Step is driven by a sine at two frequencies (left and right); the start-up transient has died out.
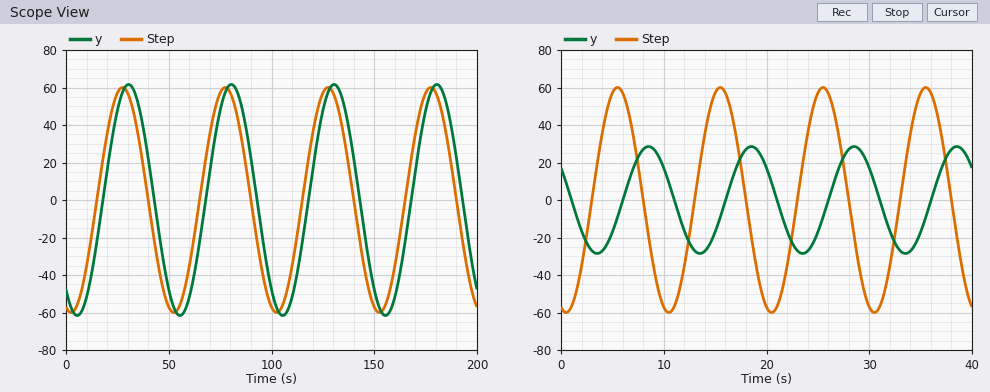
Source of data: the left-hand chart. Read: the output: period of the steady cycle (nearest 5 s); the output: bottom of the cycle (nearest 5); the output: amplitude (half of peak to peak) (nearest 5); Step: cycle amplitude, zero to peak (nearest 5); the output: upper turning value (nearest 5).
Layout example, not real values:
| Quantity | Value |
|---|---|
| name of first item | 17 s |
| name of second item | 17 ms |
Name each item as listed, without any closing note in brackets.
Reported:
| Quantity | Value |
|---|---|
| the output: period of the steady cycle | 50 s |
| the output: bottom of the cycle | -60 |
| the output: amplitude (half of peak to peak) | 60 |
| Step: cycle amplitude, zero to peak | 60 |
| the output: upper turning value | 60 |
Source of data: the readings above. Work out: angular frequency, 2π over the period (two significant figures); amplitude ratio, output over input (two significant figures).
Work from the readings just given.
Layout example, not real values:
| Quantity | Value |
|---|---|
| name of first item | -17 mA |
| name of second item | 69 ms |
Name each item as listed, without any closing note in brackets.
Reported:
| Quantity | Value |
|---|---|
| angular frequency, 2π over the period | 0.13 rad/s |
| amplitude ratio, output over input | 1.0 |
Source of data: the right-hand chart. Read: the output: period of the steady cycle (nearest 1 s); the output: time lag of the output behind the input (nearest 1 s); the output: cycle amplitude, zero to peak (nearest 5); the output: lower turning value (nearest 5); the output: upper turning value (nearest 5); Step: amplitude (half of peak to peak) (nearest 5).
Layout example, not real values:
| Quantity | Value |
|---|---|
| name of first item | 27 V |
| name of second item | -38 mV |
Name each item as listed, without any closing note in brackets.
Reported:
| Quantity | Value |
|---|---|
| the output: period of the steady cycle | 10 s |
| the output: time lag of the output behind the input | 3 s |
| the output: cycle amplitude, zero to peak | 30 |
| the output: lower turning value | -30 |
| the output: upper turning value | 30 |
| Step: amplitude (half of peak to peak) | 60 |
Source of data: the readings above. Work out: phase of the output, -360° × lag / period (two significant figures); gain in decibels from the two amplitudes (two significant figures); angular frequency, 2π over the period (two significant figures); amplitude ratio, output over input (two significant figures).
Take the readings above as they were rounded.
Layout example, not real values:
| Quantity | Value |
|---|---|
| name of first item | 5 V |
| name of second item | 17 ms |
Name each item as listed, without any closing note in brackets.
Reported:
| Quantity | Value |
|---|---|
| phase of the output, -360° × lag / period | -110° |
| gain in decibels from the two amplitudes | -6.0 dB |
| angular frequency, 2π over the period | 0.63 rad/s |
| amplitude ratio, output over input | 0.50 |
